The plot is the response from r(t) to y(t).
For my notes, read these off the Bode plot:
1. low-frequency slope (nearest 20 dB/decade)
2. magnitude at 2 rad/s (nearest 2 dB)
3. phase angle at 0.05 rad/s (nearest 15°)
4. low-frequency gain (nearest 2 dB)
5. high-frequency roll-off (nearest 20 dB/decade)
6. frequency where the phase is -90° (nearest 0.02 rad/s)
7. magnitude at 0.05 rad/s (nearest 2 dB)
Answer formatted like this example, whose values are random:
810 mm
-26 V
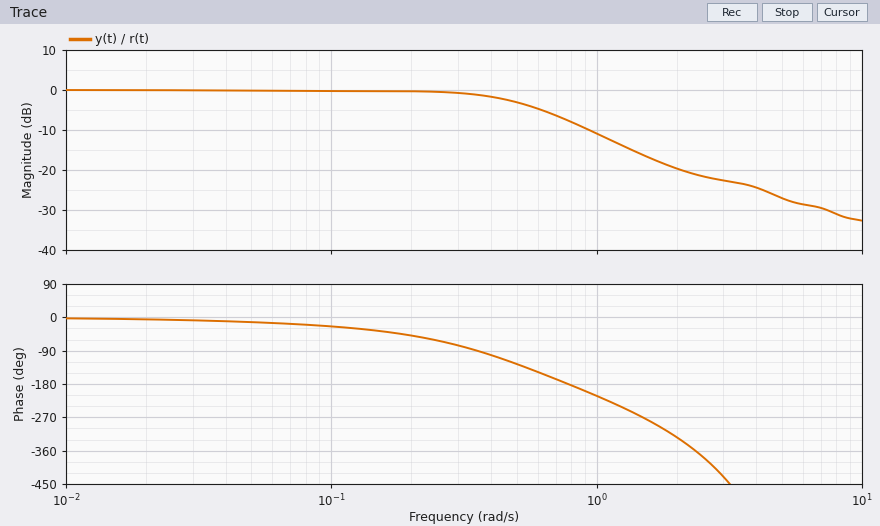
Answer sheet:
0 dB/decade
-20 dB
-15°
0 dB
-20 dB/decade
0.36 rad/s
0 dB
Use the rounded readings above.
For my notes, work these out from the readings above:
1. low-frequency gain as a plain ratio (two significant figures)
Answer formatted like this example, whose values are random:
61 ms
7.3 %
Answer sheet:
1.0
